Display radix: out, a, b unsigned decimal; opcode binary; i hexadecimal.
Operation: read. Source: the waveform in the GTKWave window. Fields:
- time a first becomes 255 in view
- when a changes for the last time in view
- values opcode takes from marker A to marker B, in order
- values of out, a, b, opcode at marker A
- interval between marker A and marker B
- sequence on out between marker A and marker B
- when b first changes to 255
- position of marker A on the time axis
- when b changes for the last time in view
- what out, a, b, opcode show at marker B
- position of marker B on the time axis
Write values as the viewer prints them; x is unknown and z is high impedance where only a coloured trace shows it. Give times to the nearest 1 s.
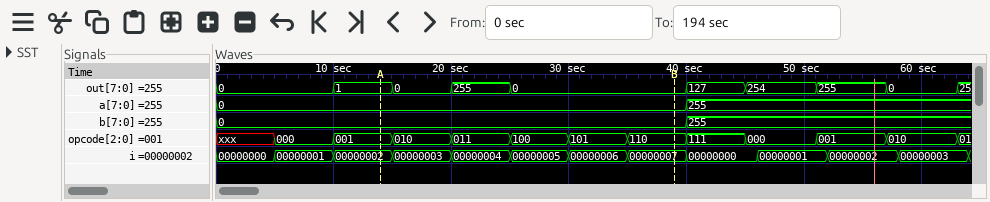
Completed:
40 s
40 s
001, 010, 011, 100, 101, 110
out=1, a=0, b=0, opcode=001
25 s
1, 0, 255, 0
40 s
14 s
40 s
out=0, a=0, b=0, opcode=110
39 s
